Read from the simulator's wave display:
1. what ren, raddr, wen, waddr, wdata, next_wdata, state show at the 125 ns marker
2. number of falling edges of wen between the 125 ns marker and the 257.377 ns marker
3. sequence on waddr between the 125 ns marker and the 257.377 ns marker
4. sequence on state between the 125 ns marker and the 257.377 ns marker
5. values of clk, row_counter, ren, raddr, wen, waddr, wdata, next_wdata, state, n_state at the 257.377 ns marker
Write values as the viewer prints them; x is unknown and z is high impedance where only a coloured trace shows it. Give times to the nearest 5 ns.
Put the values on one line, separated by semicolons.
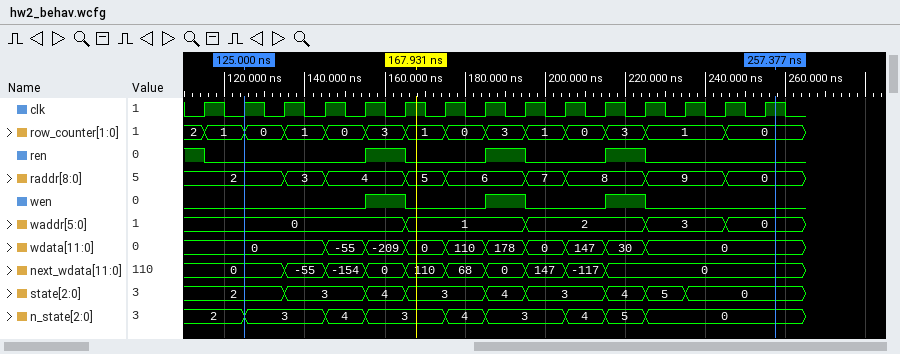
ren=0, raddr=2, wen=0, waddr=0, wdata=0, next_wdata=0, state=2; 3; 0, 1, 2, 3, 0; 2, 3, 4, 3, 4, 3, 4, 5, 0; clk=1, row_counter=0, ren=0, raddr=0, wen=0, waddr=0, wdata=0, next_wdata=0, state=0, n_state=0
